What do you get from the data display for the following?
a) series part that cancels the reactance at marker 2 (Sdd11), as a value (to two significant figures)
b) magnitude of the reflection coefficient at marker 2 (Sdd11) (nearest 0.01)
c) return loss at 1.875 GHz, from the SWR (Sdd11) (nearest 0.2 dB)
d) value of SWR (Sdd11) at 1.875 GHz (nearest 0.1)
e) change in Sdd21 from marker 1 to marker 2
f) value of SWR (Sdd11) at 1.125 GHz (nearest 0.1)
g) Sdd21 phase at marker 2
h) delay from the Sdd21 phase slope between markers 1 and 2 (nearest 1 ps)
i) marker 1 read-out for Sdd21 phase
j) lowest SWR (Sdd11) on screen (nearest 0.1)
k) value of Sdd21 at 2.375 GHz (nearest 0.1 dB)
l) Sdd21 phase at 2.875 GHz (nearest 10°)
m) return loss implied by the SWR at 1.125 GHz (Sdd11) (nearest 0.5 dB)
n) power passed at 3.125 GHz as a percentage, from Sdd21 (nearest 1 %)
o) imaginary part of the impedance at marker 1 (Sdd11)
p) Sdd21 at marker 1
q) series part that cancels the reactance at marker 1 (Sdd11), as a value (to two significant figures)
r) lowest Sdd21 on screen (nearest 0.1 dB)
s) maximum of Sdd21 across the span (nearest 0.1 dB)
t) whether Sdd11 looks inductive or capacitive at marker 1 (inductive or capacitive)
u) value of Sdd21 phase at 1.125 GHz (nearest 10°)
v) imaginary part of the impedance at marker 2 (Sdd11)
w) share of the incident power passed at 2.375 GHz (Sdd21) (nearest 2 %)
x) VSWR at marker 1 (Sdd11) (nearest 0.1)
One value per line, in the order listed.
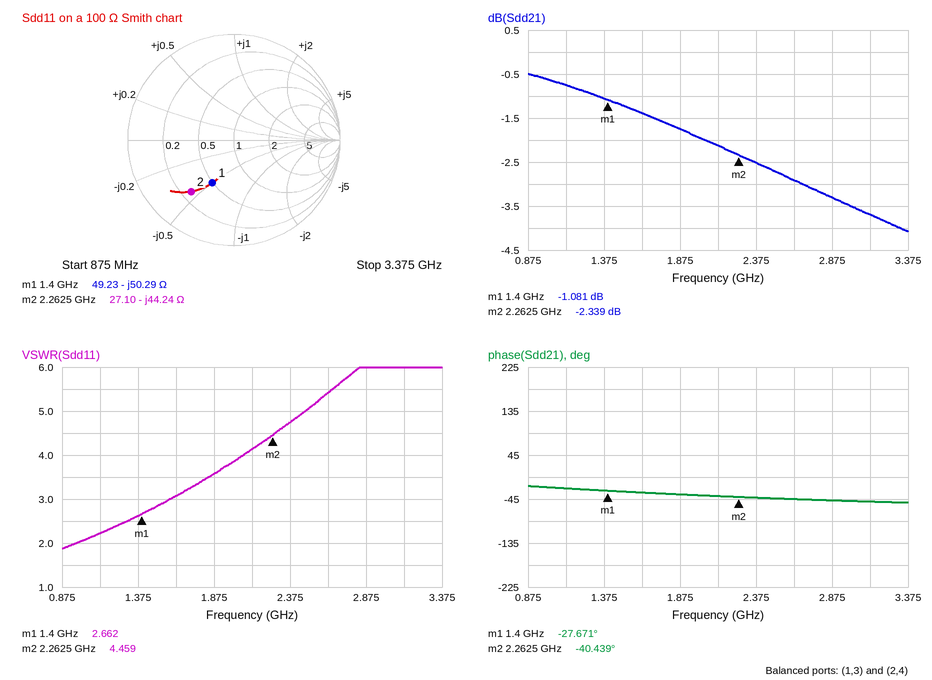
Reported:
3.1 nH
0.63
5.0 dB
3.6
-1.258 dB
2.2
-40.439°
41 ps
-27.671°
1.9
-2.5 dB
-50°
8.5 dB
43 %
-50.29 Ω
-1.081 dB
5.7 nH
-4.1 dB
-0.5 dB
capacitive
-20°
-44.24 Ω
56 %
2.7
